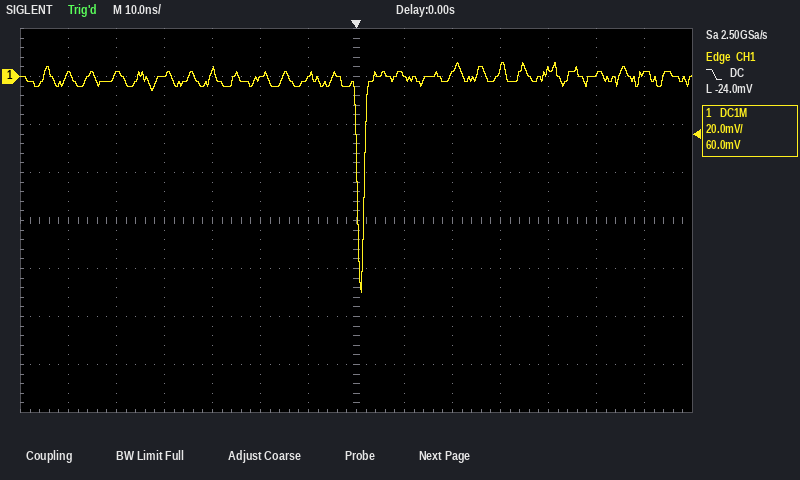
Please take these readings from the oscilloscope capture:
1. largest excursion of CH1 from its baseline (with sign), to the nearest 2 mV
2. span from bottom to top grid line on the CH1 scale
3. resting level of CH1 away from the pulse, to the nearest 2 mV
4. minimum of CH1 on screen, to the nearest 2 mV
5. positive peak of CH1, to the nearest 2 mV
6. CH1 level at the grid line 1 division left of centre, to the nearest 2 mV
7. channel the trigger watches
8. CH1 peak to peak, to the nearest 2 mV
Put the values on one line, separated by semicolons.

-90 mV; 160 mV; 0 mV; -90 mV; 6 mV; 0 mV; CH1; 96 mV
